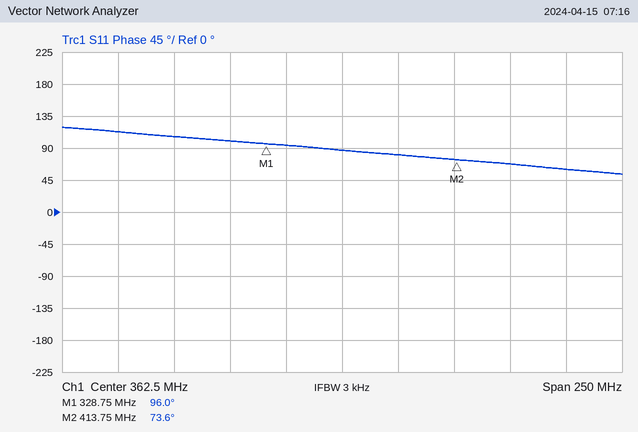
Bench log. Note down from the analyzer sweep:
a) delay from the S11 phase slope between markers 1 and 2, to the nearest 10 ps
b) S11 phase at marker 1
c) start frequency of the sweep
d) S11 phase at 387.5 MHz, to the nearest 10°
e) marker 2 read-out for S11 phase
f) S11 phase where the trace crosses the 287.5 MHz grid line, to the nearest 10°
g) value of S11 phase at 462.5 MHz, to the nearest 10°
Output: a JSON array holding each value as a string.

["730 ps", "96.0°", "237.5 MHz", "80°", "73.6°", "110°", "60°"]
